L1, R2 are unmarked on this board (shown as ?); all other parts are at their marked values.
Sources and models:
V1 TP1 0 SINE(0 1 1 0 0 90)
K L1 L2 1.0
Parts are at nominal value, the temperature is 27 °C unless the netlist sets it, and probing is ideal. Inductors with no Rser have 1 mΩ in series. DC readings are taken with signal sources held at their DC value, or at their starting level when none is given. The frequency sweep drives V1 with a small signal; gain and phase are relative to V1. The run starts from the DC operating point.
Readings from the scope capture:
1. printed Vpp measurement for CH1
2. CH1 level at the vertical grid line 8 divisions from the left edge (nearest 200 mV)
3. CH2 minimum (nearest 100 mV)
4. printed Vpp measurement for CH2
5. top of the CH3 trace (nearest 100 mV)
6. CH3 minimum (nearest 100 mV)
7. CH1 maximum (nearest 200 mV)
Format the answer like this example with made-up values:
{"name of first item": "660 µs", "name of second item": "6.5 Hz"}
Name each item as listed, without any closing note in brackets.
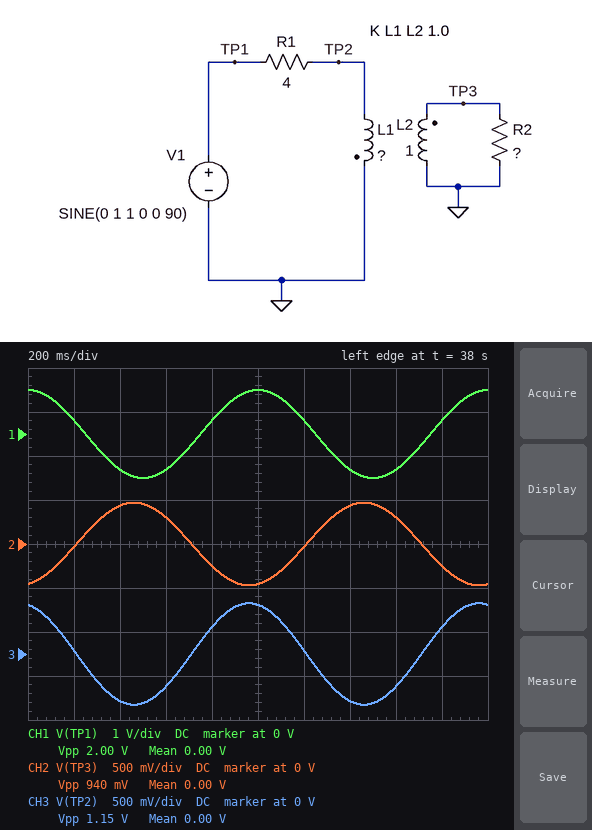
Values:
{"printed Vpp measurement for CH1": "2.00 V", "CH1 level at the vertical grid line 8 divisions from the left edge": "-800 mV", "CH2 minimum": "-500 mV", "printed Vpp measurement for CH2": "940 mV", "top of the CH3 trace": "600 mV", "CH3 minimum": "-600 mV", "CH1 maximum": "1.0 V"}
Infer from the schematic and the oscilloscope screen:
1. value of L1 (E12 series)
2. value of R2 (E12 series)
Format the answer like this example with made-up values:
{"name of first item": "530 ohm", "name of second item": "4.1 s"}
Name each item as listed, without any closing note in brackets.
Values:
{"value of L1": "1.5 H", "value of R2": "3.9 Ω"}
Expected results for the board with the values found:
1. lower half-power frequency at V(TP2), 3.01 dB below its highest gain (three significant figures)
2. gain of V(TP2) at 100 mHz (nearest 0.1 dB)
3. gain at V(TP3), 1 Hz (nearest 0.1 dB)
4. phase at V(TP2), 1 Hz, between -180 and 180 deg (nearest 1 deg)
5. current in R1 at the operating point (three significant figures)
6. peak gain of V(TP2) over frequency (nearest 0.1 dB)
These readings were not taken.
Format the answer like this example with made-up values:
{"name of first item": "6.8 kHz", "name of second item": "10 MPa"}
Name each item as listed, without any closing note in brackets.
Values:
{"lower half-power frequency at V(TP2), 3.01 dB below its highest gain": "252 mHz", "gain of V(TP2) at 100 mHz": "-13.2 dB", "gain at V(TP3), 1 Hz": "-6.6 dB", "phase at V(TP2), 1 Hz, between -180 and 180 deg": "14 deg", "current in R1 at the operating point": "250 mA", "peak gain of V(TP2) over frequency": "-4.5 dB"}
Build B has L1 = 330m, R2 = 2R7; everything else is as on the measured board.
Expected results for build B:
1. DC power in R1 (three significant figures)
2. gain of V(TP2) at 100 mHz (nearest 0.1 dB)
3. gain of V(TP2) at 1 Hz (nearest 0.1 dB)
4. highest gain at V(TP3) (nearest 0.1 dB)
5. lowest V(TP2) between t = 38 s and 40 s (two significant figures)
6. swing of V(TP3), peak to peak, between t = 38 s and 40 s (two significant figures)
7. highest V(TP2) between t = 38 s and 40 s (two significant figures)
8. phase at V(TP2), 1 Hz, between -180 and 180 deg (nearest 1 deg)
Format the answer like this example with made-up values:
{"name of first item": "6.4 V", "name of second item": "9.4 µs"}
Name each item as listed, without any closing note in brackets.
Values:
{"DC power in R1": "250 mW", "gain of V(TP2) at 100 mHz": "-26.0 dB", "gain of V(TP2) at 1 Hz": "-15.3 dB", "highest gain at V(TP3)": "-10.0 dB", "lowest V(TP2) between t = 38 s and 40 s": "-170 mV", "swing of V(TP3), peak to peak, between t = 38 s and 40 s": "600 mV", "highest V(TP2) between t = 38 s and 40 s": "170 mV", "phase at V(TP2), 1 Hz, between -180 and 180 deg": "19 deg"}
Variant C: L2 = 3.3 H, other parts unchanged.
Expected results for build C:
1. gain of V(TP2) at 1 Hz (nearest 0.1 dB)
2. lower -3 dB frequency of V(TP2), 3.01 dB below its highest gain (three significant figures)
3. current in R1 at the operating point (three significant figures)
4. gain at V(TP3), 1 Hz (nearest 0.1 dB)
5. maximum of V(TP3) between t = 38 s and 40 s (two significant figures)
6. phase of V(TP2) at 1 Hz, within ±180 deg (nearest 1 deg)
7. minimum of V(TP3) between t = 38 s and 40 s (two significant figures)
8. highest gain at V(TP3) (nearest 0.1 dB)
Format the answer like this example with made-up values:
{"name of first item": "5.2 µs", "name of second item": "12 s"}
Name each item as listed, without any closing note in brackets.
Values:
{"gain of V(TP2) at 1 Hz": "-10.3 dB", "lower -3 dB frequency of V(TP2), 3.01 dB below its highest gain": "130 mHz", "current in R1 at the operating point": "250 mA", "gain at V(TP3), 1 Hz": "-6.9 dB", "maximum of V(TP3) between t = 38 s and 40 s": "450 mV", "phase of V(TP2) at 1 Hz, within ±180 deg": "7 deg", "minimum of V(TP3) between t = 38 s and 40 s": "-450 mV", "highest gain at V(TP3)": "-6.8 dB"}
